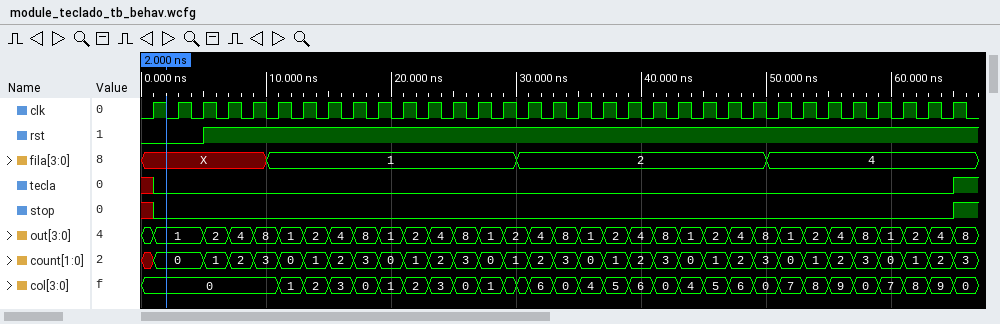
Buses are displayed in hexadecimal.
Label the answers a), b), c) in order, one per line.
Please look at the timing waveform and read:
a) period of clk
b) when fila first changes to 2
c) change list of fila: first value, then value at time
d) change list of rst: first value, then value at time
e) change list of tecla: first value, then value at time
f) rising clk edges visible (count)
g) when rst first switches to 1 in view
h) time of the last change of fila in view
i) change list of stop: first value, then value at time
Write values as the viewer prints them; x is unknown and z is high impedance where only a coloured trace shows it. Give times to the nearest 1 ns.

a) 2 ns
b) 30 ns
c) X, 1 at 10 ns, 2 at 30 ns, 4 at 50 ns
d) 0, 1 at 5 ns
e) x, 0 at 1 ns, 1 at 65 ns
f) 33
g) 5 ns
h) 50 ns
i) x, 0 at 1 ns, 1 at 65 ns
